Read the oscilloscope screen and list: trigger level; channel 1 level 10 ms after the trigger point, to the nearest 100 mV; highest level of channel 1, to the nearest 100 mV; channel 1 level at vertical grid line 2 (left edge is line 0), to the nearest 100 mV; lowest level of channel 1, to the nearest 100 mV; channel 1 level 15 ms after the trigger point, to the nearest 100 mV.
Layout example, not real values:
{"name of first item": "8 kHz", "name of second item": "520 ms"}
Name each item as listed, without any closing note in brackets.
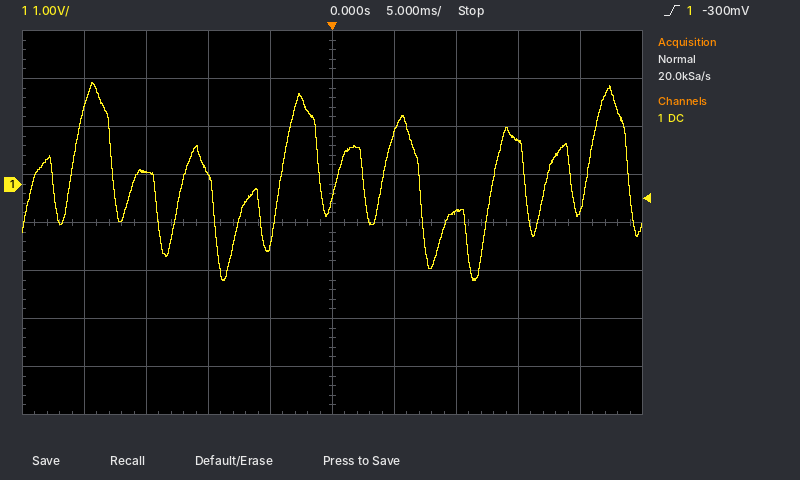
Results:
{"trigger level": "-300 mV", "channel 1 level 10 ms after the trigger point, to the nearest 100 mV": "-600 mV", "highest level of channel 1, to the nearest 100 mV": "2.1 V", "channel 1 level at vertical grid line 2 (left edge is line 0), to the nearest 100 mV": "300 mV", "lowest level of channel 1, to the nearest 100 mV": "-2.0 V", "channel 1 level 15 ms after the trigger point, to the nearest 100 mV": "900 mV"}
